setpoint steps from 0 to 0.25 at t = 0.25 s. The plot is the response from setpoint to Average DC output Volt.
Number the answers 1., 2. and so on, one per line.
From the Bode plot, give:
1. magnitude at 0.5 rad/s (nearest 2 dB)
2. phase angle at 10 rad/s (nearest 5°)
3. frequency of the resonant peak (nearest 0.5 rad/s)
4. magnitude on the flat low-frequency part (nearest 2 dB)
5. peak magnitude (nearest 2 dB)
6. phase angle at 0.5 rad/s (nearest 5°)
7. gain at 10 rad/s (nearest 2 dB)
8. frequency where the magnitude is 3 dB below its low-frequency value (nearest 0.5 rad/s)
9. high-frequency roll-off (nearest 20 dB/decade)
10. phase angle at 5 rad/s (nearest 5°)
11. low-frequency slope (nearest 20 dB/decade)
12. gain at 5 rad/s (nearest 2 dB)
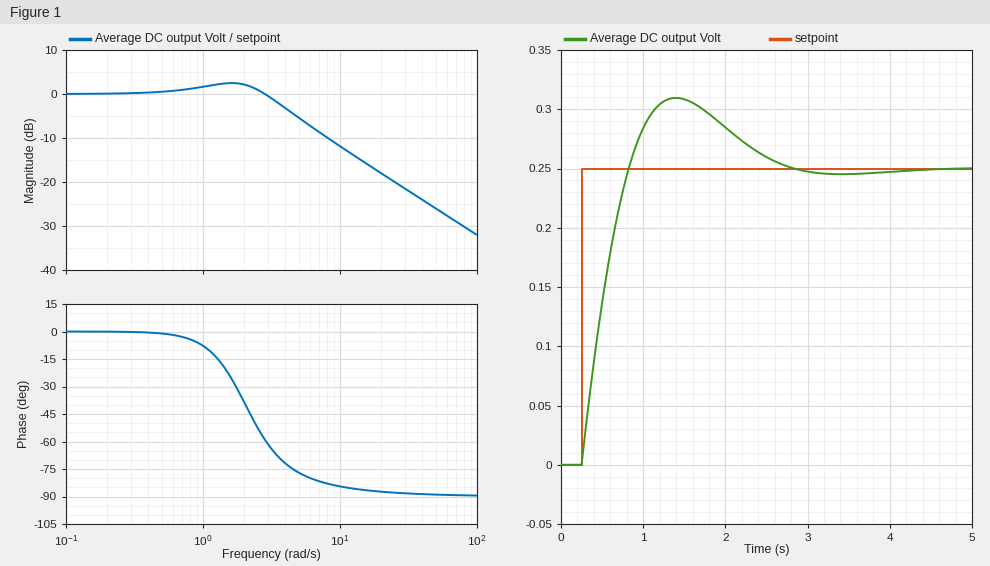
1. 0 dB
2. -85°
3. 1.5 rad/s
4. 0 dB
5. 2 dB
6. 0°
7. -12 dB
8. 4.0 rad/s
9. -20 dB/decade
10. -75°
11. 0 dB/decade
12. -6 dB
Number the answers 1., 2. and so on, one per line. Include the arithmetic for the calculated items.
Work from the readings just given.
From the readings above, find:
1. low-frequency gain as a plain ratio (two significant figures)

1. 10^(0 / 20) = 1.0
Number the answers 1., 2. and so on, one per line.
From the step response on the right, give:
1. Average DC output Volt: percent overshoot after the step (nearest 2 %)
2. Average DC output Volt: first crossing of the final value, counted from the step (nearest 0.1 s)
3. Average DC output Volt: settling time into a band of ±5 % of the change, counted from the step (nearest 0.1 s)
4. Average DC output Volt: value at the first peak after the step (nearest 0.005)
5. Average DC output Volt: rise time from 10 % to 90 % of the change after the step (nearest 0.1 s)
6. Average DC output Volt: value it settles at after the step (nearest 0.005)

1. 24 %
2. 0.6 s
3. 2.2 s
4. 0.310
5. 0.4 s
6. 0.250
